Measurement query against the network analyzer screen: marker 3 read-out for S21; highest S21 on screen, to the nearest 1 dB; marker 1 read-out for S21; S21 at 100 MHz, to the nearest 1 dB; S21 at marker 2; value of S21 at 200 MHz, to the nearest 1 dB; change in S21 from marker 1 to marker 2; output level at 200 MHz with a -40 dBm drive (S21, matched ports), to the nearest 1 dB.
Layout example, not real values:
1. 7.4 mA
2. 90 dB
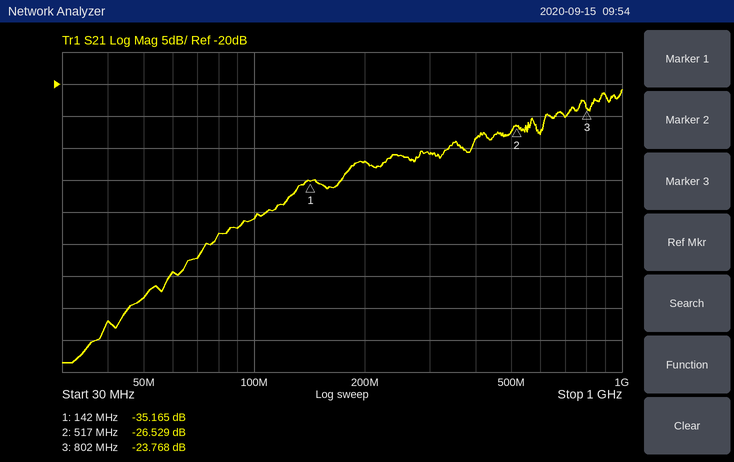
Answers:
1. -23.768 dB
2. -21 dB
3. -35.165 dB
4. -41 dB
5. -26.529 dB
6. -32 dB
7. 8.636 dB
8. -72 dBm
